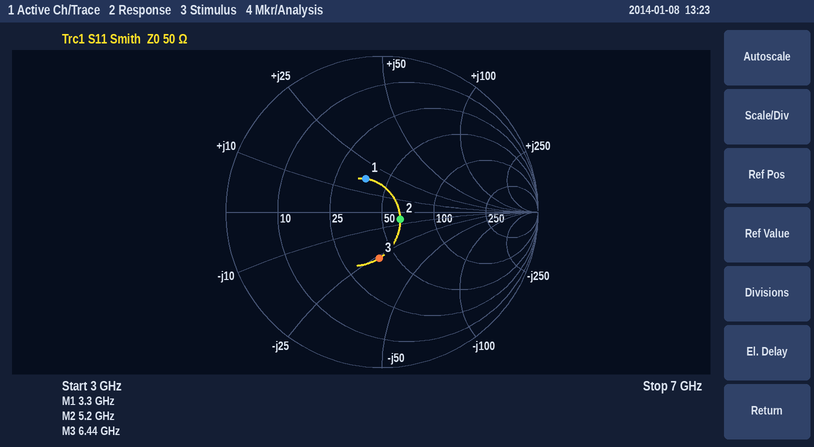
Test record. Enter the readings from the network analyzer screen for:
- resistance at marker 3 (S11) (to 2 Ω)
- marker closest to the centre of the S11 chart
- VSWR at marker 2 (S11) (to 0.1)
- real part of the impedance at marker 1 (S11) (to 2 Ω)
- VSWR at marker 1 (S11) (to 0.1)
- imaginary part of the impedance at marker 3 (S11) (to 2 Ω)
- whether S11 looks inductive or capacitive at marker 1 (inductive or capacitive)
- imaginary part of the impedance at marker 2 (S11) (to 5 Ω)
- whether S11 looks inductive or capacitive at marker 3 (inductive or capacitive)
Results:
40 Ω
marker 2
1.3
38 Ω
1.6
-26 Ω
inductive
-5 Ω
capacitive
